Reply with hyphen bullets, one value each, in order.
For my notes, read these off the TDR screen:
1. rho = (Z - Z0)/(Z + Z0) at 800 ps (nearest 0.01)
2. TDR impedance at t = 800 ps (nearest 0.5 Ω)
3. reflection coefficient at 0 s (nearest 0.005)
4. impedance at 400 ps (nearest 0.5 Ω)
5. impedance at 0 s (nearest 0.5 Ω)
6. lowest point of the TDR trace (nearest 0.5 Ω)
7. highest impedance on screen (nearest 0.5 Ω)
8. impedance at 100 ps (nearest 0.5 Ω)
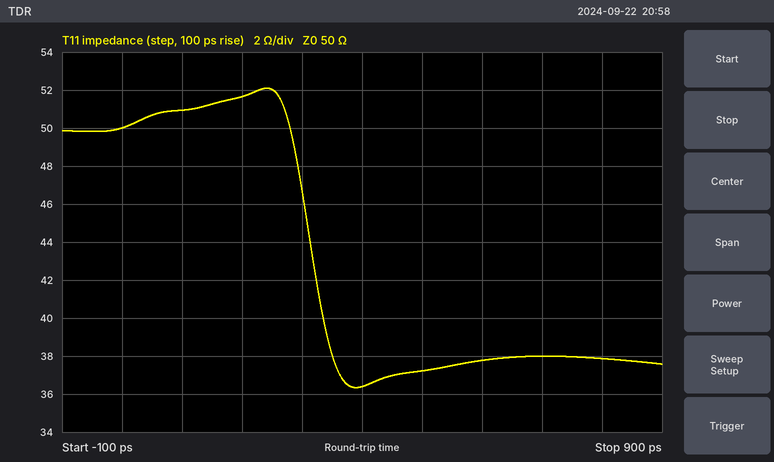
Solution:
- -0.14
- 38.0 Ω
- 0.000
- 36.5 Ω
- 50.0 Ω
- 36.5 Ω
- 52.0 Ω
- 51.0 Ω
